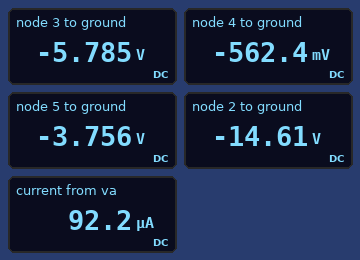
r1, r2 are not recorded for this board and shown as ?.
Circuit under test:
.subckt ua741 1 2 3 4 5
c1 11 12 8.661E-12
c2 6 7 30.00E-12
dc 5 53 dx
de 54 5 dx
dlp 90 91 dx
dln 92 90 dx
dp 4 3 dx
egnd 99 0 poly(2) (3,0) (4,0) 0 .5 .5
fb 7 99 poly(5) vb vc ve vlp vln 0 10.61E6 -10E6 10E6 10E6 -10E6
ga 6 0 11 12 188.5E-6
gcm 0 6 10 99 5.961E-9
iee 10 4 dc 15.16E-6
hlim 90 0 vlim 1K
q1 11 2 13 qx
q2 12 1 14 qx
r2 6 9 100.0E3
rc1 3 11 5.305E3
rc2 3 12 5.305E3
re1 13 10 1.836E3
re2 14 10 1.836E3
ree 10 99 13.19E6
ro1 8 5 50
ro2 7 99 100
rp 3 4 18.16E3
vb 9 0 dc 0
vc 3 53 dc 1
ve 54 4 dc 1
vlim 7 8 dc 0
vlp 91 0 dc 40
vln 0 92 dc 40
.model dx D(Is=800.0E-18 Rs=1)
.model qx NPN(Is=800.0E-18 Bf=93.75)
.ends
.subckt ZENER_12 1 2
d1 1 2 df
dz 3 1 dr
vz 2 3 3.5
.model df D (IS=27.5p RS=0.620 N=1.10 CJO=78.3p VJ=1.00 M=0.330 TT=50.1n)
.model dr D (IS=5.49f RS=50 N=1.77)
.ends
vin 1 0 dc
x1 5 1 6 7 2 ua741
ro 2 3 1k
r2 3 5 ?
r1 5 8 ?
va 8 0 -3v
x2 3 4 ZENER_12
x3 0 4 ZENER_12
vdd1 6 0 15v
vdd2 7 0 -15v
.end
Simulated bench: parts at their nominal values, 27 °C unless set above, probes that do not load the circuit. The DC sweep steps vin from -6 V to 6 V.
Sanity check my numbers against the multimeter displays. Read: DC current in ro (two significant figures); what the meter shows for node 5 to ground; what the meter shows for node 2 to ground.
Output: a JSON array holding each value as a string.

["8.8 mA", "-3.756 V", "-14.61 V"]
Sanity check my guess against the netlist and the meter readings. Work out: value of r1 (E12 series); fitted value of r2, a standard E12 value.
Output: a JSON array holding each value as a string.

["8.2 kΩ", "22 kΩ"]
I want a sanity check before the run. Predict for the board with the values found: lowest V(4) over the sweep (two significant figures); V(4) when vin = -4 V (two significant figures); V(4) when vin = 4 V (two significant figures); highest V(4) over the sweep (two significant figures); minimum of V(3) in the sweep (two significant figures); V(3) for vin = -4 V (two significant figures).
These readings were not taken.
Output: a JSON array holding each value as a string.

["-560 mV", "5.2 V", "-560 mV", "5.2 V", "-5.8 V", "5.8 V"]
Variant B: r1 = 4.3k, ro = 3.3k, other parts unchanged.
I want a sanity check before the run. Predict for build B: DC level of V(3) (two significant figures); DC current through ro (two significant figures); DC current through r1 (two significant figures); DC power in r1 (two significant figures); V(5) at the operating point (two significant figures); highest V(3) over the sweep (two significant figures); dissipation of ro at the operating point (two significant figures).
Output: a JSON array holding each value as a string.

["-5.4 V", "2.8 mA", "91 µA", "36 µW", "-3.4 V", "5.4 V", "26 mW"]
